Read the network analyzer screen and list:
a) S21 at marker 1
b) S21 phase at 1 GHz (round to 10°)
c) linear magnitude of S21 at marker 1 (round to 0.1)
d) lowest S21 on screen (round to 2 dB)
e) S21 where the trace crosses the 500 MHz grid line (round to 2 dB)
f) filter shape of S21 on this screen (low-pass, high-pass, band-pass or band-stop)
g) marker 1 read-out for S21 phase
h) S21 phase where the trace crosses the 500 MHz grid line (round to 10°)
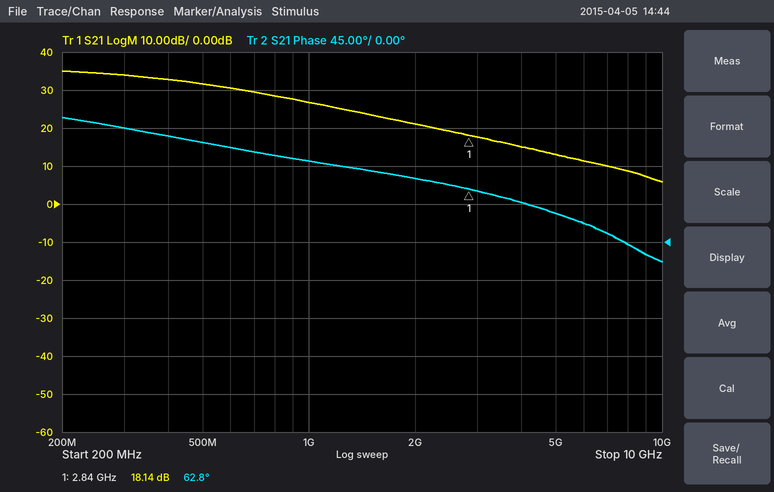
18.14 dB
100°
8.1
6 dB
32 dB
low-pass
62.8°
120°
